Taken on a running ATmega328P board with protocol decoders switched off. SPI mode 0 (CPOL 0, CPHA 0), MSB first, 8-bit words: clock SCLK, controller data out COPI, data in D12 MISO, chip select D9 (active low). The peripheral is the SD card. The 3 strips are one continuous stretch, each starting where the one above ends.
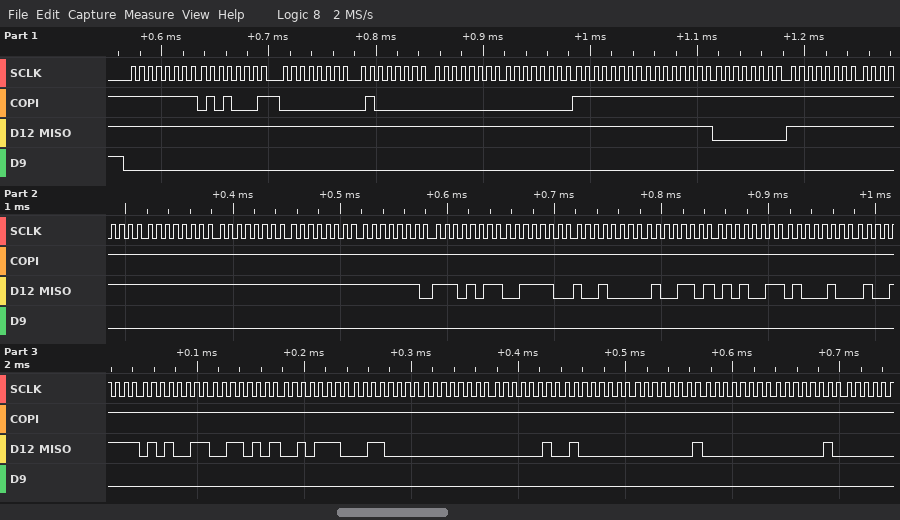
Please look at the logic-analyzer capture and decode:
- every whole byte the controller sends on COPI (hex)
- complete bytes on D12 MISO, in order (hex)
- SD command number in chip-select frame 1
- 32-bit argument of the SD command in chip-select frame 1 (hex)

FF 51 00 40 00 00 FF FF FF FF FF FF FF FF FF FF FF FF FF FF FF FF FF FF FF FF FF FF FF FF FF FF
FF FF FF FF FF FF FF FF 00 FF FF FF FF FF FE EB 3C 90 4D 53 44 4F 53 35 2E 30 00 02 40 01 00 02
CMD17
0x00400000
